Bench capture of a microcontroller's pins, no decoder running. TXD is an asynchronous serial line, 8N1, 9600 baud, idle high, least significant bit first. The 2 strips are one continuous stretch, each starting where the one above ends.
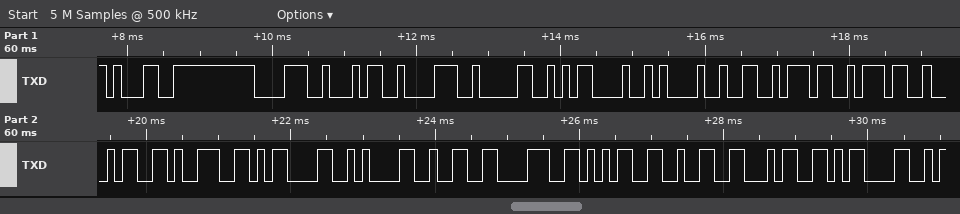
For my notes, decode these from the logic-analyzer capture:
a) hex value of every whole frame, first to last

31 38 34 38 30 0D 0A 32 37 37 34 39 0D 0A 32 38 35 32 34 0D
